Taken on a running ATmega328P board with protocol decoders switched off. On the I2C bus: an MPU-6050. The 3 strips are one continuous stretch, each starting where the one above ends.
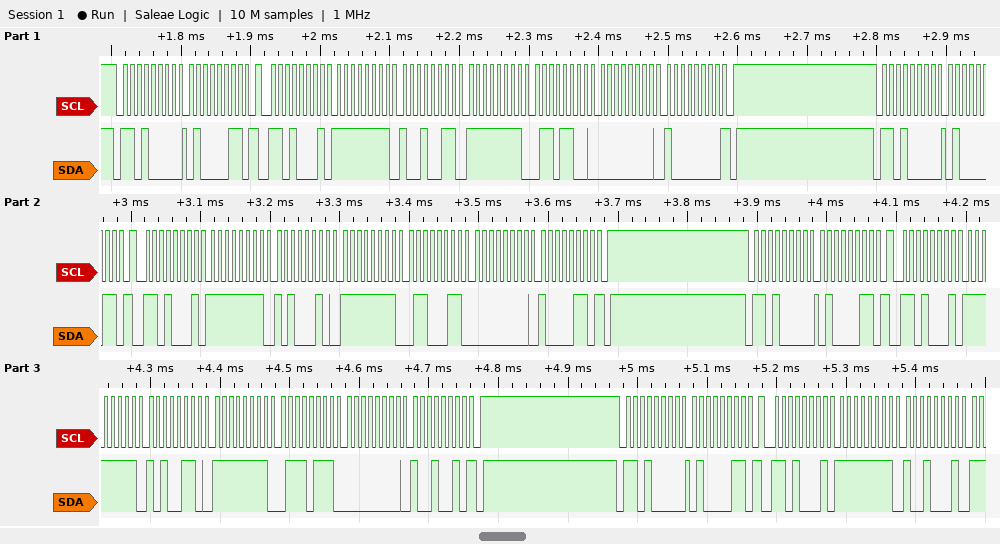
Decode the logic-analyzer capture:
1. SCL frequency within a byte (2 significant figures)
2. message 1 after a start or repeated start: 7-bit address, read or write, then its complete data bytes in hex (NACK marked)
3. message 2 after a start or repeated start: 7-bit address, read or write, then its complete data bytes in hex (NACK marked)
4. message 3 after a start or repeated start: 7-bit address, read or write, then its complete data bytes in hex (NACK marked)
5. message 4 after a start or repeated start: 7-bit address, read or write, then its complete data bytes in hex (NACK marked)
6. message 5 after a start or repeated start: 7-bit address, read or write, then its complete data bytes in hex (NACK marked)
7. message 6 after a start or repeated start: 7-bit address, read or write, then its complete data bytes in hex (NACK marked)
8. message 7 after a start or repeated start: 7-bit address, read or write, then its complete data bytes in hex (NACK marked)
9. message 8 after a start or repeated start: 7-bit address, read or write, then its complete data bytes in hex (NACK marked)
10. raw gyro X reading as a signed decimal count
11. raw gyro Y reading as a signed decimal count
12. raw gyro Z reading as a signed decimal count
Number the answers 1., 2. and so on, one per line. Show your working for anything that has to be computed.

1. 100 kHz
2. 0x68 write: 43
3. 0x68 read: FF 93 FF 6C 00 80 NACK
4. 0x68 write: 43
5. 0x68 read: FF A2 FF 63 00 86 NACK
6. 0x68 write: 43
7. 0x68 read: FF A6 FF 77 00 92 NACK
8. 0x68 write: 43
9. 0x68 read: FF 91
10. 0xFF93 = -109
11. 0xFF6C = -148
12. 0x0080 = 128
